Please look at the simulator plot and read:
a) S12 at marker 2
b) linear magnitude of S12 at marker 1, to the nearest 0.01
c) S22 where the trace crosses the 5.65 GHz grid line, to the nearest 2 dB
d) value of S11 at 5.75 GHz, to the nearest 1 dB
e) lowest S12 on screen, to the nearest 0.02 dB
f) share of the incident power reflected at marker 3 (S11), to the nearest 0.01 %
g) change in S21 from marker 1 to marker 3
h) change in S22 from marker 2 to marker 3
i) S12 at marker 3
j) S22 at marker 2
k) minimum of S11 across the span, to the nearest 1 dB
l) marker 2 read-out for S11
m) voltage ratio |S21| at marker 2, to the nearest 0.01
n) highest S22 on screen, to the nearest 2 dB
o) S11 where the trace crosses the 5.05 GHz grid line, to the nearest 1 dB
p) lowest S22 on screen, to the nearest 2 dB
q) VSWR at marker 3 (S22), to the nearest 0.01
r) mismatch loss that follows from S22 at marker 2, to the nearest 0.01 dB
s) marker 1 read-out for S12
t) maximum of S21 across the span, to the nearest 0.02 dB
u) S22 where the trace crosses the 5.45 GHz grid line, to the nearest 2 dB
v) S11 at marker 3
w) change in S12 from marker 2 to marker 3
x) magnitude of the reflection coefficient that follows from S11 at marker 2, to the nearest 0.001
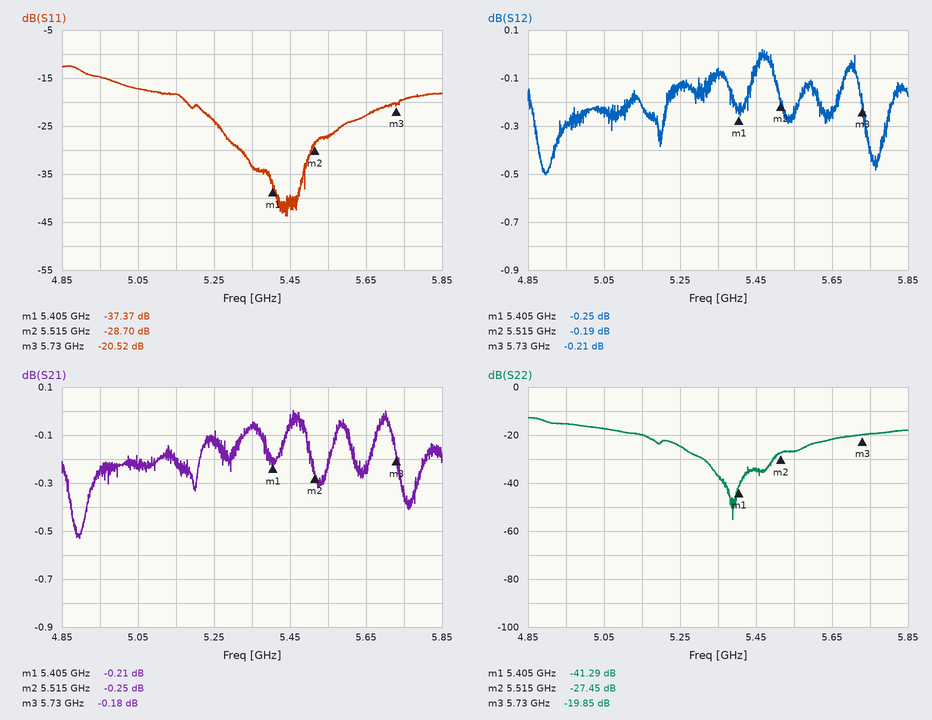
-0.19 dB
0.97
-22 dB
-19 dB
-0.50 dB
0.89 %
0.03 dB
7.60 dB
-0.21 dB
-27.45 dB
-44 dB
-28.70 dB
0.97
-12 dB
-17 dB
-56 dB
1.23
0.01 dB
-0.25 dB
0.00 dB
-34 dB
-20.52 dB
-0.02 dB
0.037
